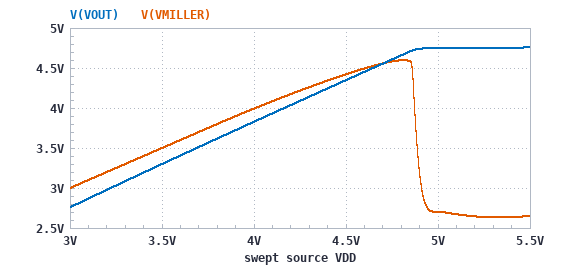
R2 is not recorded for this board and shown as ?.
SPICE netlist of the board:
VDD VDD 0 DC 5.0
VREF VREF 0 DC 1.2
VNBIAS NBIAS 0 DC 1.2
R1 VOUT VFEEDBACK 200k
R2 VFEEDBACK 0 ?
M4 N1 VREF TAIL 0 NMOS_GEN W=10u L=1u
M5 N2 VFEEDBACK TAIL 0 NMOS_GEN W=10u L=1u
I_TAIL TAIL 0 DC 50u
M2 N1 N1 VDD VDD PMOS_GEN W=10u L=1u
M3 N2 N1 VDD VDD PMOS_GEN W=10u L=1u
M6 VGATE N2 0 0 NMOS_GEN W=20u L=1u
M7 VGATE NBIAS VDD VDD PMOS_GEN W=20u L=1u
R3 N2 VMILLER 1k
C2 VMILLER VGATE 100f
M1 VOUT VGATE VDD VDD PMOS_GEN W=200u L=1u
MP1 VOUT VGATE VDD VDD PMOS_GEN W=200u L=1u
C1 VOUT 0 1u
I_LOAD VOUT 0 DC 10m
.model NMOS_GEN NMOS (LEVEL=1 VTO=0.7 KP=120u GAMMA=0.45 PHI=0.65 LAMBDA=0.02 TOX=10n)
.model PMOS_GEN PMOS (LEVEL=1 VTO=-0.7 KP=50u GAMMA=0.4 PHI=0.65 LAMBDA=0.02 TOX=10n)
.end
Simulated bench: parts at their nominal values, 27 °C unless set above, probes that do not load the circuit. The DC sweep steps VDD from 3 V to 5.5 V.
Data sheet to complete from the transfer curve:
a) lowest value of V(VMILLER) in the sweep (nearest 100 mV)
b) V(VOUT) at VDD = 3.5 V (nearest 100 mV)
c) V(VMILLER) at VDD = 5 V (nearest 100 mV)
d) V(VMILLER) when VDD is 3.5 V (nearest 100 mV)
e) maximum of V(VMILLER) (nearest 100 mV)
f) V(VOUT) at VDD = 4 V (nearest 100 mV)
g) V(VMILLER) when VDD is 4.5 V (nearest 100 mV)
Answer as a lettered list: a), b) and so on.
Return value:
a) 2.6 V
b) 3.3 V
c) 2.7 V
d) 3.5 V
e) 4.6 V
f) 3.8 V
g) 4.4 V
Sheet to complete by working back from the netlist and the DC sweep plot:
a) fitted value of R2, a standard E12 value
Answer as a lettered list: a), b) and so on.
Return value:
a) 68 kΩ
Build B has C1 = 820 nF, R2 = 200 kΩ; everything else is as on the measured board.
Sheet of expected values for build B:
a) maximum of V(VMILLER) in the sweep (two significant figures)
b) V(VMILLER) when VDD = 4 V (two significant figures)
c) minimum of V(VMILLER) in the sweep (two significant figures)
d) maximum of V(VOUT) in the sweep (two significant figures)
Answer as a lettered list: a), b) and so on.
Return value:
a) 2.6 V
b) 2.0 V
c) 1.4 V
d) 2.4 V
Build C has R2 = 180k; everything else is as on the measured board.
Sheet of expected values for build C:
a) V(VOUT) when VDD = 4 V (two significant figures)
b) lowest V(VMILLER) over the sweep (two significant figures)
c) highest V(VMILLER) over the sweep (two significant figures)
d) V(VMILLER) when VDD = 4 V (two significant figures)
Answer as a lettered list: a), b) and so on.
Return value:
a) 2.5 V
b) 1.4 V
c) 2.6 V
d) 2.0 V
